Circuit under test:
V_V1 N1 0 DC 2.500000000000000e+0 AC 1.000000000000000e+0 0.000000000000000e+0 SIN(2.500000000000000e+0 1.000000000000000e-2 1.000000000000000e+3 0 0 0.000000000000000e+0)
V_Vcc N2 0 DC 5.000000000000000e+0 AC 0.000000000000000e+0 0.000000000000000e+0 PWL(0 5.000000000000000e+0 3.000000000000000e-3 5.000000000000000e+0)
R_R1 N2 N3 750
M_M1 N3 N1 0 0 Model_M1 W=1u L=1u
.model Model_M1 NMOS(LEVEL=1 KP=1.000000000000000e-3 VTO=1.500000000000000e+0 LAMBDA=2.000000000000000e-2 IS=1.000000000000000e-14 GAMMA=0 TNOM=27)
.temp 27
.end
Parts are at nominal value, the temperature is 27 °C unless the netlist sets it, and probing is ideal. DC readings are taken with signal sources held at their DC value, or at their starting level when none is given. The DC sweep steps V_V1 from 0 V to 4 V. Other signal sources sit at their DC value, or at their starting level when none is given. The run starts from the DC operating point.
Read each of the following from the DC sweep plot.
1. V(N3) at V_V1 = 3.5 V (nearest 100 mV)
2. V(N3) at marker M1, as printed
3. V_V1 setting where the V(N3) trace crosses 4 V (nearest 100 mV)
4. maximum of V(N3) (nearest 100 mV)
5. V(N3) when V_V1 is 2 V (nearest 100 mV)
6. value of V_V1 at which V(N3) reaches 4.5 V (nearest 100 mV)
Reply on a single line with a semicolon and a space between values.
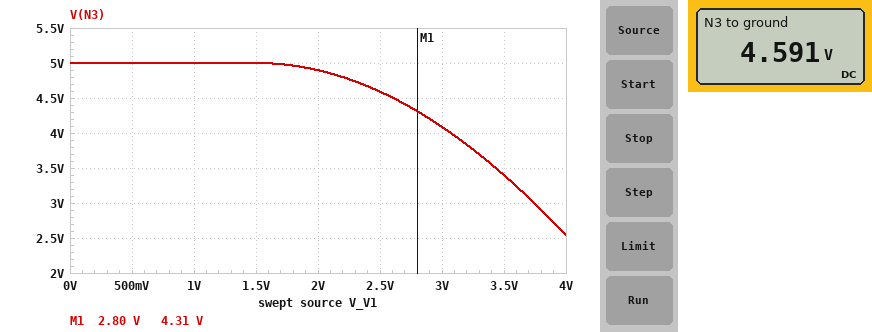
3.4 V; 4.31 V; 3.1 V; 5.0 V; 4.9 V; 2.6 V
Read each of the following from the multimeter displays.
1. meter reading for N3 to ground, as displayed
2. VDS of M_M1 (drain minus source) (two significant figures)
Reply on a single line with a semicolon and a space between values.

4.591 V; 4.6 V
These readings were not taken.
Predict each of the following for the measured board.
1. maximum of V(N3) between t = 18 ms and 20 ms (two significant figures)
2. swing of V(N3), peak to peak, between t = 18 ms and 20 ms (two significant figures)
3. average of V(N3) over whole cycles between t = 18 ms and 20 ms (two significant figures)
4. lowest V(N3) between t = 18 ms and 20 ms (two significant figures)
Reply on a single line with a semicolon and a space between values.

4.6 V; 16 mV; 4.6 V; 4.6 V
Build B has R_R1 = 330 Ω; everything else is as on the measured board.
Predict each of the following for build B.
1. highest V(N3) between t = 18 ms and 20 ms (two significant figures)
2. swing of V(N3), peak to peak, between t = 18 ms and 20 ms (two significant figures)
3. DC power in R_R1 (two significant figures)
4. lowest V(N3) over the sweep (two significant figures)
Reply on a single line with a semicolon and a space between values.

4.8 V; 7.2 mV; 99 µW; 3.9 V
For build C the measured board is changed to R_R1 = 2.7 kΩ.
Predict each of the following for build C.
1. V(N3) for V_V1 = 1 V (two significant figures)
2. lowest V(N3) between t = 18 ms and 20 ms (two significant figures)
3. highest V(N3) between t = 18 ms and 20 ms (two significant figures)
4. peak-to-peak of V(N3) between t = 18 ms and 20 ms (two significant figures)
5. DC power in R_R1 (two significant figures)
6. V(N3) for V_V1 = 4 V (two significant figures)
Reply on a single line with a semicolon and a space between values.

5.0 V; 3.5 V; 3.6 V; 56 mV; 770 µW; 730 mV
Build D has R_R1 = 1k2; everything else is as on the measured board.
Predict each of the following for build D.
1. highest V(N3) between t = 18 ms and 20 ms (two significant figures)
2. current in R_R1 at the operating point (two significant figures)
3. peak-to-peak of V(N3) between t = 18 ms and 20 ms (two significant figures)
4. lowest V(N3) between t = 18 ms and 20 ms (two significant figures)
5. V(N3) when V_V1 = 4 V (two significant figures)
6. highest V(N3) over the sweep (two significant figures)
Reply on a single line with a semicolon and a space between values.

4.4 V; 540 µA; 26 mV; 4.3 V; 1.6 V; 5.0 V
